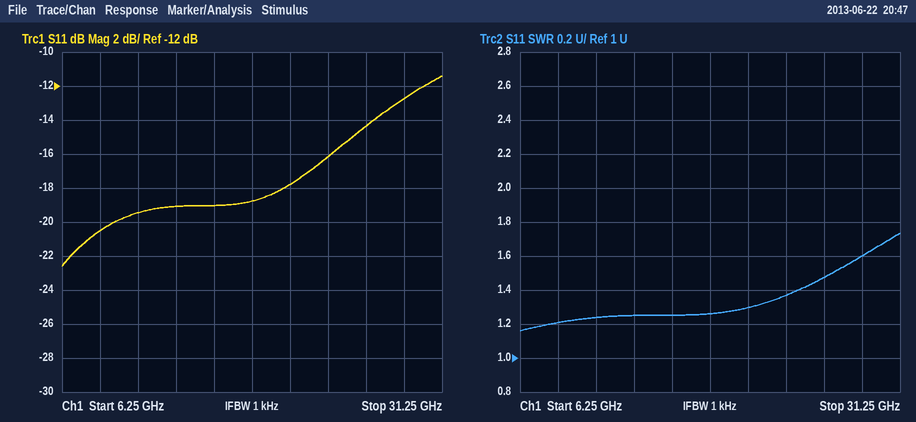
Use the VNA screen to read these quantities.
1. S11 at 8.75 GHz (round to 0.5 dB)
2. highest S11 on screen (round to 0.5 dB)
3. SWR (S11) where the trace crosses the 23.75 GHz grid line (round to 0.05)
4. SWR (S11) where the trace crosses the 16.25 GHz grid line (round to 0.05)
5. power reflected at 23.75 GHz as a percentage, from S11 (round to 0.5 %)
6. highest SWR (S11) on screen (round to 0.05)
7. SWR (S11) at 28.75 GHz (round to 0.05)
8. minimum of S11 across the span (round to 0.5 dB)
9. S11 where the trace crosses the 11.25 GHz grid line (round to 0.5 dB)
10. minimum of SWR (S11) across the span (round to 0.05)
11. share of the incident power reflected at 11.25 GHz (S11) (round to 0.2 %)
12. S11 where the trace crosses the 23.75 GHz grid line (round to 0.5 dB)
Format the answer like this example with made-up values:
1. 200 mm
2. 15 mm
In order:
1. -20.5 dB
2. -11.5 dB
3. 1.35
4. 1.25
5. 2.5 %
6. 1.75
7. 1.60
8. -22.5 dB
9. -19.5 dB
10. 1.15
11. 1.2 %
12. -16.0 dB
